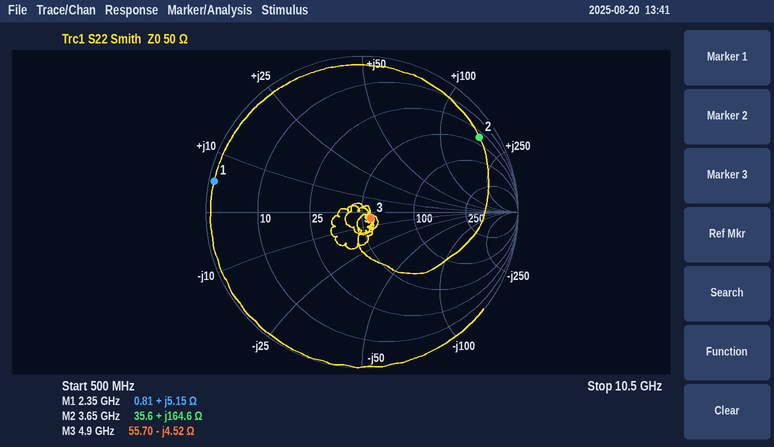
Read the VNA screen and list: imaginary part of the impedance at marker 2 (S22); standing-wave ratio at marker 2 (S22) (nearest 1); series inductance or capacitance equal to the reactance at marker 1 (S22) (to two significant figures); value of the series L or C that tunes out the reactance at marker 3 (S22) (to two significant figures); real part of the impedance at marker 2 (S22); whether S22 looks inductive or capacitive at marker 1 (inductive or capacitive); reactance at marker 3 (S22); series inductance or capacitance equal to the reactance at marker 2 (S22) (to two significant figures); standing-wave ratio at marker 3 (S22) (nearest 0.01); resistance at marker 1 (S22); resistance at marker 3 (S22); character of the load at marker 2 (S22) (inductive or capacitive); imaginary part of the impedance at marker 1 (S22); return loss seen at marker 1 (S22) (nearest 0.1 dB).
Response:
+164.6 Ω
17
350 pH
150 pH
35.6 Ω
inductive
-4.52 Ω
7.2 nH
1.15
0.81 Ω
55.70 Ω
inductive
+5.15 Ω
0.3 dB
